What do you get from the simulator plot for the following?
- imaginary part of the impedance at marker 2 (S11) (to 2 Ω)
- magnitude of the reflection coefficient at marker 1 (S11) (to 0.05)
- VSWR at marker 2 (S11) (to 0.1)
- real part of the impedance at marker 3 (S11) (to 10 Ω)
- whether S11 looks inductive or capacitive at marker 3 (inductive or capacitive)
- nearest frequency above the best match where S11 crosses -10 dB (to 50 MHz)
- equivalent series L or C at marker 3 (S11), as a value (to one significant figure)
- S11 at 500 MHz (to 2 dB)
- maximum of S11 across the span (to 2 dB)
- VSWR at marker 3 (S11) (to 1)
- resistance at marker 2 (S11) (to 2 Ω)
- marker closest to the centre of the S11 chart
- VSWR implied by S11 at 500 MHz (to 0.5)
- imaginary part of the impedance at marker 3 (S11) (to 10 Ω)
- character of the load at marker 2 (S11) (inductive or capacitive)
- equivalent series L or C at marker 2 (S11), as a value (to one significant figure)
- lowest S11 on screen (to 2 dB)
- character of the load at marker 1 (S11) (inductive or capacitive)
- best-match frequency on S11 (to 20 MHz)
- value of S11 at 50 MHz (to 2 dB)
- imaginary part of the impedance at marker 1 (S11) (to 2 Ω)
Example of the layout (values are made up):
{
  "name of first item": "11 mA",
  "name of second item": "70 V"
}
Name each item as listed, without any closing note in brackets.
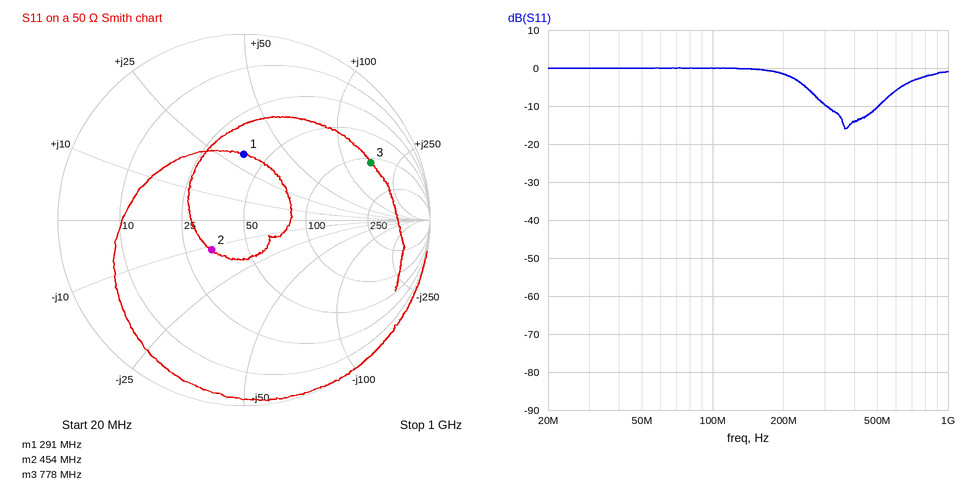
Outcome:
{
  "imaginary part of the impedance at marker 2 (S11)": "-12 Ω",
  "magnitude of the reflection coefficient at marker 1 (S11)": "0.35",
  "VSWR at marker 2 (S11)": "1.6",
  "real part of the impedance at marker 3 (S11)": "110 Ω",
  "whether S11 looks inductive or capacitive at marker 3": "inductive",
  "nearest frequency above the best match where S11 crosses -10 dB": "500 MHz",
  "equivalent series L or C at marker 3 (S11), as a value": "30 nH",
  "S11 at 500 MHz": "-10 dB",
  "maximum of S11 across the span": "0 dB",
  "VSWR at marker 3 (S11)": "7",
  "resistance at marker 2 (S11)": "34 Ω",
  "marker closest to the centre of the S11 chart": "marker 2",
  "VSWR implied by S11 at 500 MHz": "2.0",
  "imaginary part of the impedance at marker 3 (S11)": "+160 Ω",
  "character of the load at marker 2 (S11)": "capacitive",
  "equivalent series L or C at marker 2 (S11), as a value": "30 pF",
  "lowest S11 on screen": "-16 dB",
  "character of the load at marker 1 (S11)": "inductive",
  "best-match frequency on S11": "360 MHz",
  "value of S11 at 50 MHz": "0 dB",
  "imaginary part of the impedance at marker 1 (S11)": "+32 Ω"
}
